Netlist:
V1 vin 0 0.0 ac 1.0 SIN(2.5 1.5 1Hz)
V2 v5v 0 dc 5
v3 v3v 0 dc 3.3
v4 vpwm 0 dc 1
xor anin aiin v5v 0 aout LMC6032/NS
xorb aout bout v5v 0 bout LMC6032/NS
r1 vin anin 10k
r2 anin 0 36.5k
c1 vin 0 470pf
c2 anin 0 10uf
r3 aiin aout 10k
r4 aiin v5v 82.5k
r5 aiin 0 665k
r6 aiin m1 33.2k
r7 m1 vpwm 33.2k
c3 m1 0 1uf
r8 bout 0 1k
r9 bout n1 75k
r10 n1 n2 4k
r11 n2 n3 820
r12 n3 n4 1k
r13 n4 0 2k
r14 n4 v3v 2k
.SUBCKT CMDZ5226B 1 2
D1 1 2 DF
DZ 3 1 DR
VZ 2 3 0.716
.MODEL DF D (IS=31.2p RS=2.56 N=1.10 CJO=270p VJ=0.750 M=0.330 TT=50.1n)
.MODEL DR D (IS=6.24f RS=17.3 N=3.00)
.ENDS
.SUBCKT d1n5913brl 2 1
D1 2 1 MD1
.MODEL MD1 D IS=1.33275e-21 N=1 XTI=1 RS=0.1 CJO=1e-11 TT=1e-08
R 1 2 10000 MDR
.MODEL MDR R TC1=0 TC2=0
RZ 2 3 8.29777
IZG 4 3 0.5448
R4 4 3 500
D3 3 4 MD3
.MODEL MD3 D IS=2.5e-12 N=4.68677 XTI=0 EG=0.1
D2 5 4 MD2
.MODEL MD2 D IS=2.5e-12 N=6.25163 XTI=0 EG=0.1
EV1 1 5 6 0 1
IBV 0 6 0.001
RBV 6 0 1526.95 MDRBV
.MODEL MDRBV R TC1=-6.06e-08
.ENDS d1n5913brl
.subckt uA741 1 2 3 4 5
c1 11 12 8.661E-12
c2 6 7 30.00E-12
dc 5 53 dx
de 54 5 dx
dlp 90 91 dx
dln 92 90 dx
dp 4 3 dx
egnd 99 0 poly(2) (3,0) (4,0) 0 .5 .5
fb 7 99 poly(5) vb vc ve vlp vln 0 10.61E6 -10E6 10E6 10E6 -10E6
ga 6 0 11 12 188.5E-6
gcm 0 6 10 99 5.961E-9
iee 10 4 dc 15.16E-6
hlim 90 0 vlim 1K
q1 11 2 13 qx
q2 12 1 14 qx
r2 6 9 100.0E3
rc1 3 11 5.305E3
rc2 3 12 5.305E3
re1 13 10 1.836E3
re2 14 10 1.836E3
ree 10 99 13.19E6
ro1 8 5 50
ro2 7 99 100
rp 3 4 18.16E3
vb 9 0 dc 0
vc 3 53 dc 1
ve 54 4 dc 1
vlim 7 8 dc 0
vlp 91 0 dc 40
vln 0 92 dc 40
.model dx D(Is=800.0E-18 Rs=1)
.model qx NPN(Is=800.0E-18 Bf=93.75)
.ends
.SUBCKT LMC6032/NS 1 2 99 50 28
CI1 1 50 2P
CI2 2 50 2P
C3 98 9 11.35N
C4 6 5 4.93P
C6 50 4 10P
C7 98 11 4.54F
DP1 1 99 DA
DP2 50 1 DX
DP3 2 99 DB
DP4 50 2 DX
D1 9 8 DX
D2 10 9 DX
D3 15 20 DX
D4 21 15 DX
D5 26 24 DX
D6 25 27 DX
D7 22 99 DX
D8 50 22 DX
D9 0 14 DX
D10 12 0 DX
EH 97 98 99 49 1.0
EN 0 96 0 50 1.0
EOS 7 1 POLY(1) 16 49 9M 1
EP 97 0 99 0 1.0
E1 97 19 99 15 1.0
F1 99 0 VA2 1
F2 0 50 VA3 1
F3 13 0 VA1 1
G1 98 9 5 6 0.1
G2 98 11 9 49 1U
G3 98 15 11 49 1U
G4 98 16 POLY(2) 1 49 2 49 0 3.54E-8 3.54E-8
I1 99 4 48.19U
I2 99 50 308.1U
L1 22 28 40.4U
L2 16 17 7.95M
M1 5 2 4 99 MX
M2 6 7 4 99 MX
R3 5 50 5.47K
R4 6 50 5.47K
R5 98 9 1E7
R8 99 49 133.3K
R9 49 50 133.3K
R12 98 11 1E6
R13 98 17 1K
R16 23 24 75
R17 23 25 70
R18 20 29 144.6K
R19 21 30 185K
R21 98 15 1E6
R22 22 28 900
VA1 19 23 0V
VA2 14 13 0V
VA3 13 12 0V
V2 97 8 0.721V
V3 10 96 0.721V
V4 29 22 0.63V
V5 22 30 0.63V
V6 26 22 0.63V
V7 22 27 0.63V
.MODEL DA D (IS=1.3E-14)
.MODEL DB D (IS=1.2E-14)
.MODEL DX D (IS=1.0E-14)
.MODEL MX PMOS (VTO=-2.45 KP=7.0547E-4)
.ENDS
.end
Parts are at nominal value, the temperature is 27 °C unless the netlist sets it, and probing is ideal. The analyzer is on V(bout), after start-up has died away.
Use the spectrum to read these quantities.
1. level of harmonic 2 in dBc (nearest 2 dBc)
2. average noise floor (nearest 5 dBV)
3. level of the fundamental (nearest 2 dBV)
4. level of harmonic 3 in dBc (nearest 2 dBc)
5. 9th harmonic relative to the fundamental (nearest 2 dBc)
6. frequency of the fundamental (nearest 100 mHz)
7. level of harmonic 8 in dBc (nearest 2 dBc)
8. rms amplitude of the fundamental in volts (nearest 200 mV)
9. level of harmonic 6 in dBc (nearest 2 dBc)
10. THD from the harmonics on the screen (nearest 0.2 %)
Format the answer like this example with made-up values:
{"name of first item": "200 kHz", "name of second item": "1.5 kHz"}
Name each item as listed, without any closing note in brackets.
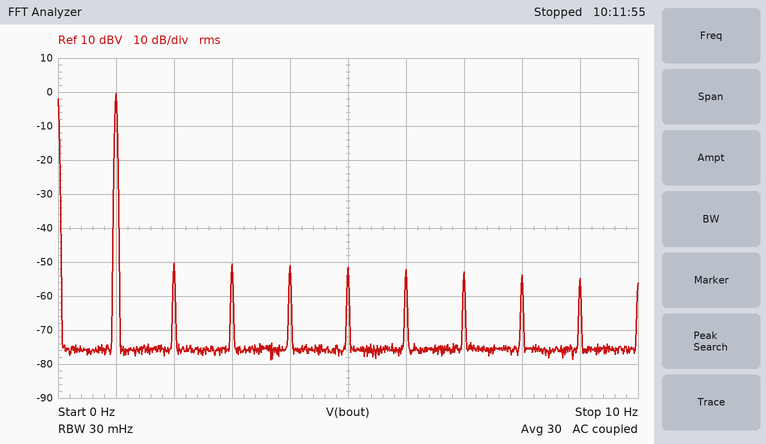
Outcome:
{"level of harmonic 2 in dBc": "-50 dBc", "average noise floor": "-75 dBV", "level of the fundamental": "0 dBV", "level of harmonic 3 in dBc": "-50 dBc", "9th harmonic relative to the fundamental": "-54 dBc", "frequency of the fundamental": "1.0 Hz", "level of harmonic 8 in dBc": "-54 dBc", "rms amplitude of the fundamental in volts": "1.0 V", "level of harmonic 6 in dBc": "-52 dBc", "THD from the harmonics on the screen": "0.8 %"}
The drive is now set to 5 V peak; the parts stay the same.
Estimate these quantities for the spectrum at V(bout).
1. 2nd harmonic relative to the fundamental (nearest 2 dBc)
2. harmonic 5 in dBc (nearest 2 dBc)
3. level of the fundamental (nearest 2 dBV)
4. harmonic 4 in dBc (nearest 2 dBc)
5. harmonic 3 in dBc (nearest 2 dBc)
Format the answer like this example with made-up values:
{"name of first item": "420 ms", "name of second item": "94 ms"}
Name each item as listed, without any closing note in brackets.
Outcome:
{"2nd harmonic relative to the fundamental": "-24 dBc", "harmonic 5 in dBc": "-20 dBc", "level of the fundamental": "2 dBV", "harmonic 4 in dBc": "-28 dBc", "harmonic 3 in dBc": "-12 dBc"}
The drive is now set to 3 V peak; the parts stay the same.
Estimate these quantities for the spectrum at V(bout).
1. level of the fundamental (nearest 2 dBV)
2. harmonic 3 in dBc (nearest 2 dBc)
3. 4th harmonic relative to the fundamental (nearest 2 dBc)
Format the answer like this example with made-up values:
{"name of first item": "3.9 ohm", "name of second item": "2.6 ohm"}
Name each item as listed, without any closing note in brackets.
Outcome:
{"level of the fundamental": "2 dBV", "harmonic 3 in dBc": "-14 dBc", "4th harmonic relative to the fundamental": "-32 dBc"}
